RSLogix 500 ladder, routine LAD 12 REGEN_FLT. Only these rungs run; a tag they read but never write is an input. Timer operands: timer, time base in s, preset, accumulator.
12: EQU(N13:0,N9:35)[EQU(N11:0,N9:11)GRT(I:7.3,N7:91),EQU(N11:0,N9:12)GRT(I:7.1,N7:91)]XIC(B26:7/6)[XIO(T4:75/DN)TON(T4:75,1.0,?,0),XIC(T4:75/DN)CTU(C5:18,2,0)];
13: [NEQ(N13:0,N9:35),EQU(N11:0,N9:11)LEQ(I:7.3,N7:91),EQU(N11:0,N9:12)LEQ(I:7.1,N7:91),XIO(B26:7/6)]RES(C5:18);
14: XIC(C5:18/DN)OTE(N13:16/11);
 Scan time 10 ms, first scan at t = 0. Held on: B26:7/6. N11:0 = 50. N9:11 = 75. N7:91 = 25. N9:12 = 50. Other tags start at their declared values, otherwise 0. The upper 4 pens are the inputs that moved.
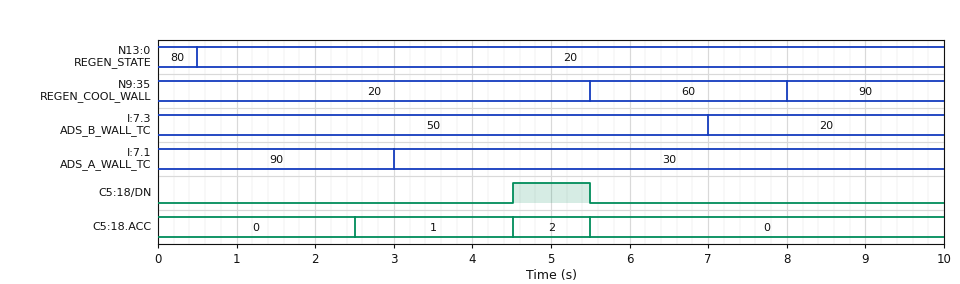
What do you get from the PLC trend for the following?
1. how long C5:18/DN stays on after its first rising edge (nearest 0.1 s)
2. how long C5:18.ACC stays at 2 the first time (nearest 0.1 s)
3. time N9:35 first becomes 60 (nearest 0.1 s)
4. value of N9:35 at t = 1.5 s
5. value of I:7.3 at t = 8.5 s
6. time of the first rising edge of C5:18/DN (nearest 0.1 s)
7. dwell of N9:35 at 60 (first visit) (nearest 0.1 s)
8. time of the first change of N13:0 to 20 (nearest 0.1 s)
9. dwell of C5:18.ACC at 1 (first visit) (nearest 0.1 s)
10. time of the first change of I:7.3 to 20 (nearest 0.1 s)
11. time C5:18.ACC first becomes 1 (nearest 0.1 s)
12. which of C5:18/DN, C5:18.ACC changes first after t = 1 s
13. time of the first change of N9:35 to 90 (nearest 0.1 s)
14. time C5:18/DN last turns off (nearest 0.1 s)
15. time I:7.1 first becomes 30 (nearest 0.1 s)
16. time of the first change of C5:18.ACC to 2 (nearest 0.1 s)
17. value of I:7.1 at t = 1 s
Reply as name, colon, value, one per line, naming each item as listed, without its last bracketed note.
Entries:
how long C5:18/DN stays on after its first rising edge: 1.0 s
how long C5:18.ACC stays at 2 the first time: 1.0 s
time N9:35 first becomes 60: 5.5 s
value of N9:35 at t = 1.5 s: 20
value of I:7.3 at t = 8.5 s: 20
time of the first rising edge of C5:18/DN: 4.5 s
dwell of N9:35 at 60 (first visit): 2.5 s
time of the first change of N13:0 to 20: 0.5 s
dwell of C5:18.ACC at 1 (first visit): 2.0 s
time of the first change of I:7.3 to 20: 7.0 s
time C5:18.ACC first becomes 1: 2.5 s
which of C5:18/DN, C5:18.ACC changes first after t = 1 s: C5:18.ACC
time of the first change of N9:35 to 90: 8.0 s
time C5:18/DN last turns off: 5.5 s
time I:7.1 first becomes 30: 3.0 s
time of the first change of C5:18.ACC to 2: 4.5 s
value of I:7.1 at t = 1 s: 90
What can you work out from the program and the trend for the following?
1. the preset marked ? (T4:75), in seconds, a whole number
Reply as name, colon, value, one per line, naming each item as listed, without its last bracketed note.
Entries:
the preset marked ? (T4:75), in seconds, a whole number: 2 s
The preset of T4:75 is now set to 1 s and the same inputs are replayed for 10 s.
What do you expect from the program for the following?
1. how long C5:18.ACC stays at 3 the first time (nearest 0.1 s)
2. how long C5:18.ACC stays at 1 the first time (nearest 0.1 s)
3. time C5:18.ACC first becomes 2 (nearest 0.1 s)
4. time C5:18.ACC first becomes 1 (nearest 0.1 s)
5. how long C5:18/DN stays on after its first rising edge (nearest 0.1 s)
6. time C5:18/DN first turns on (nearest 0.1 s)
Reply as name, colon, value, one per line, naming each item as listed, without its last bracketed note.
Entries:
how long C5:18.ACC stays at 3 the first time: 1.0 s
how long C5:18.ACC stays at 1 the first time: 1.0 s
time C5:18.ACC first becomes 2: 2.5 s
time C5:18.ACC first becomes 1: 1.5 s
how long C5:18/DN stays on after its first rising edge: 3.0 s
time C5:18/DN first turns on: 2.5 s
